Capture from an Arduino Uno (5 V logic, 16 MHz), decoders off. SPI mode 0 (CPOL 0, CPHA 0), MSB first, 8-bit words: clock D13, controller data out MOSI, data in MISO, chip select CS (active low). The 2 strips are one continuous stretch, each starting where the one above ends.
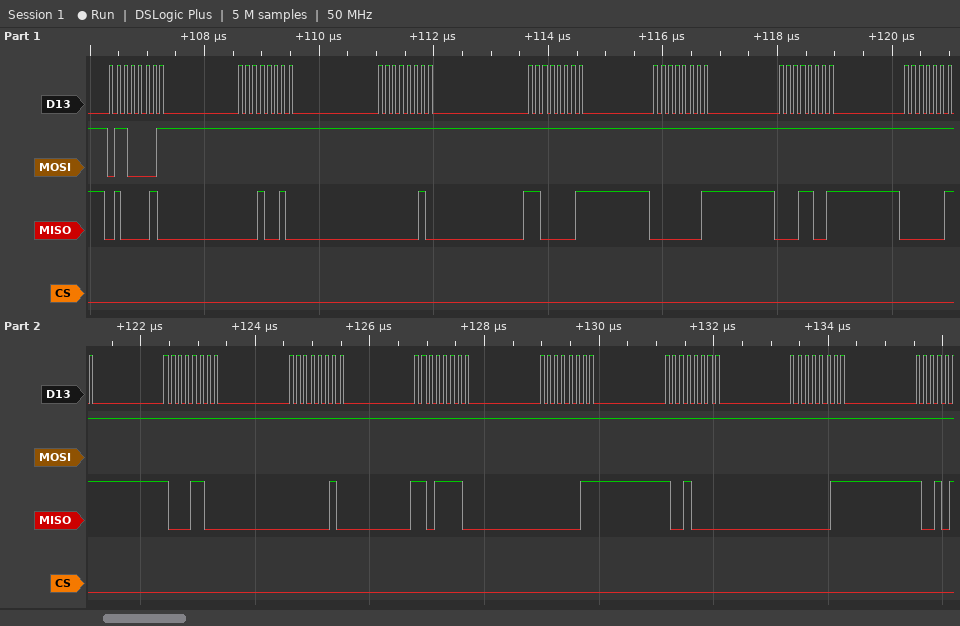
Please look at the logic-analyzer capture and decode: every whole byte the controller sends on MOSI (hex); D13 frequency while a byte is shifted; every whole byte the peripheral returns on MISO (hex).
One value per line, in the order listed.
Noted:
61 FF FF FF FF FF FF FF FF FF FF FF FF
8 MHz
42 12 02 C1 01 19 03 8C 02 DE 03 90 03
